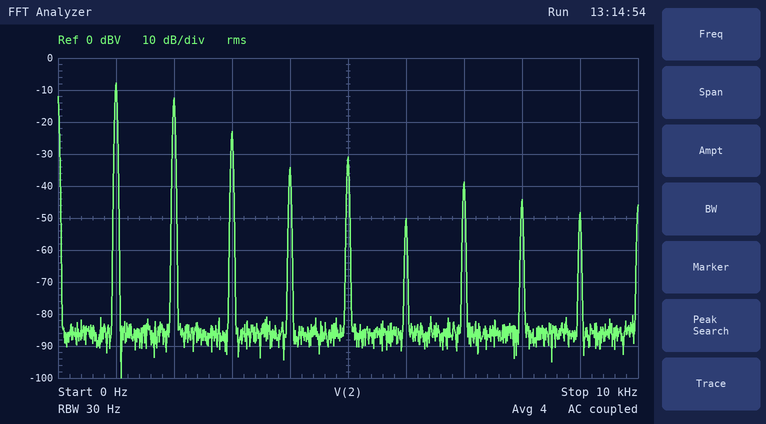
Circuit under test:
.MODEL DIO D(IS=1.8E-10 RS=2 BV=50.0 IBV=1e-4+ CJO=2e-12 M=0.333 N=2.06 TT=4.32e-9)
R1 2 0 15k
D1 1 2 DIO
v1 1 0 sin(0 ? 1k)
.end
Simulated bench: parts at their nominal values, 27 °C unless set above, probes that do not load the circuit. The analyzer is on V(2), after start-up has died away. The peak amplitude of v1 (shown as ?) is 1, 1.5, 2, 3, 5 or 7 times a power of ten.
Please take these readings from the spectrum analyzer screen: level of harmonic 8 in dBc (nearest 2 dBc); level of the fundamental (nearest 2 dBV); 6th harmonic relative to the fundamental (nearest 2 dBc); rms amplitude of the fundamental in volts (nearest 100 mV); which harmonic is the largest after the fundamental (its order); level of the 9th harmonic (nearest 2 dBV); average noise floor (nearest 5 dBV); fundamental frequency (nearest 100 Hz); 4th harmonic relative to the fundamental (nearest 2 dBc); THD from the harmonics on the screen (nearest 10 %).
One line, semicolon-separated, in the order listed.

-36 dBc; -8 dBV; -42 dBc; 400 mV; 2; -48 dBV; -85 dBV; 1.0 kHz; -26 dBc; 60 %
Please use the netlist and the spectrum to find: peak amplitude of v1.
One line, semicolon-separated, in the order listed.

2 V
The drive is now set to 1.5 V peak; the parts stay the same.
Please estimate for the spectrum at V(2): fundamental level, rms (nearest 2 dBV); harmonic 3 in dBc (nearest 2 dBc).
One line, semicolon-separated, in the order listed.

-12 dBV; -12 dBc
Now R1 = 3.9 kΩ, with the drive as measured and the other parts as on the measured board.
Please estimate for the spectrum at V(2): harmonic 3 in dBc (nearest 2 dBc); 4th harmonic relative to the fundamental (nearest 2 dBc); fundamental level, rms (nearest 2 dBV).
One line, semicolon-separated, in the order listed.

-14 dBc; -30 dBc; -8 dBV
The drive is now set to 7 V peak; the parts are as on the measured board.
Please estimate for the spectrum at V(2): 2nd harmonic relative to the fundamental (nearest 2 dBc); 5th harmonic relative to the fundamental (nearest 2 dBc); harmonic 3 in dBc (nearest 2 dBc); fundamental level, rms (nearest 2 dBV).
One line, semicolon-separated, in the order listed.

-6 dBc; -32 dBc; -26 dBc; 6 dBV
